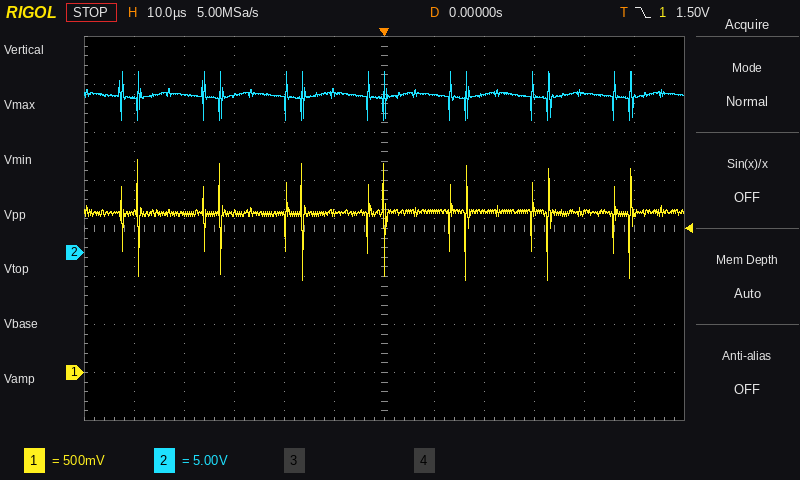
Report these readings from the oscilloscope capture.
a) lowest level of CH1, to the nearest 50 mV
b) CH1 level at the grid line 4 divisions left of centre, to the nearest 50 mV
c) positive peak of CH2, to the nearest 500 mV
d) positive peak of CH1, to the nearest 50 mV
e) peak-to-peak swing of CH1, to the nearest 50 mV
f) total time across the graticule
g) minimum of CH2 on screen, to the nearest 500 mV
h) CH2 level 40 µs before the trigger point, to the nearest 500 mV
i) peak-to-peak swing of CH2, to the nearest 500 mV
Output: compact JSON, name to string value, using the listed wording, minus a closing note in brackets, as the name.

{"lowest level of CH1, to the nearest 50 mV": "950 mV", "CH1 level at the grid line 4 divisions left of centre, to the nearest 50 mV": "1.65 V", "positive peak of CH2, to the nearest 500 mV": "19.0 V", "positive peak of CH1, to the nearest 50 mV": "2.20 V", "peak-to-peak swing of CH1, to the nearest 50 mV": "1.25 V", "total time across the graticule": "120 µs", "minimum of CH2 on screen, to the nearest 500 mV": "14.0 V", "CH2 level 40 µs before the trigger point, to the nearest 500 mV": "16.5 V", "peak-to-peak swing of CH2, to the nearest 500 mV": "5.0 V"}
